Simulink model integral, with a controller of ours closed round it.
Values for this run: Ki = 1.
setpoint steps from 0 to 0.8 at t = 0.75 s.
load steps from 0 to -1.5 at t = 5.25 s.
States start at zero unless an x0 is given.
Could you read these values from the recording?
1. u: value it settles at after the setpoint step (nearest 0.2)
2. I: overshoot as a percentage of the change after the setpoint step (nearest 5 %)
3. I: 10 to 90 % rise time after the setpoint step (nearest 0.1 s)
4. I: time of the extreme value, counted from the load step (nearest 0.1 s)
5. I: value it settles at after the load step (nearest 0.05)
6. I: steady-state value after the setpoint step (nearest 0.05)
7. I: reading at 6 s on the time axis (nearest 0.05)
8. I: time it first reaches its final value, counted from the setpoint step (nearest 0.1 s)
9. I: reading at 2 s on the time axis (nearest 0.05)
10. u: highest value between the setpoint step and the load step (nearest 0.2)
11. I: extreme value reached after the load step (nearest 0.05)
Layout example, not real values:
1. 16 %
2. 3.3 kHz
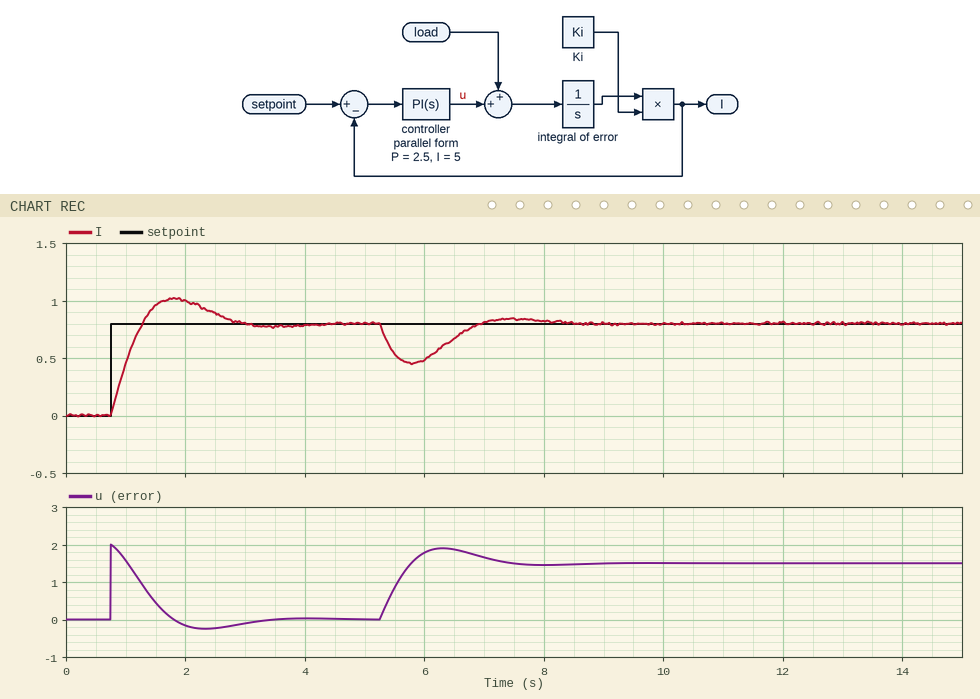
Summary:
1. 0.0
2. 25 %
3. 0.4 s
4. 0.5 s
5. 0.80
6. 0.80
7. 0.50
8. 0.5 s
9. 1.00
10. 2.0
11. 0.45
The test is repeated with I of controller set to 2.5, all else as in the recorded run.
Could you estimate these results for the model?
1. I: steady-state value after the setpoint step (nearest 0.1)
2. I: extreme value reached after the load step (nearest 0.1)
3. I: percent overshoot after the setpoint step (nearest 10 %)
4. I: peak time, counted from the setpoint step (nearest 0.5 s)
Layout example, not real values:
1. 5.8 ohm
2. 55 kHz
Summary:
1. 0.8
2. 0.4
3. 20 %
4. 1.5 s
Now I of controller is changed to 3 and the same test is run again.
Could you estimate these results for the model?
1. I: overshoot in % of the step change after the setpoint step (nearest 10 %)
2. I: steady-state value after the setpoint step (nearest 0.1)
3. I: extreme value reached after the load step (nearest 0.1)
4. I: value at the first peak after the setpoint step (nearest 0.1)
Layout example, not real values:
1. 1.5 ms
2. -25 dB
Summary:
1. 20 %
2. 0.8
3. 0.4
4. 1.0
